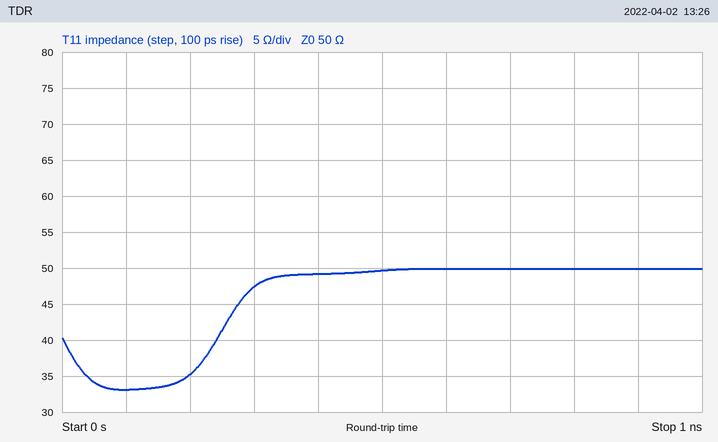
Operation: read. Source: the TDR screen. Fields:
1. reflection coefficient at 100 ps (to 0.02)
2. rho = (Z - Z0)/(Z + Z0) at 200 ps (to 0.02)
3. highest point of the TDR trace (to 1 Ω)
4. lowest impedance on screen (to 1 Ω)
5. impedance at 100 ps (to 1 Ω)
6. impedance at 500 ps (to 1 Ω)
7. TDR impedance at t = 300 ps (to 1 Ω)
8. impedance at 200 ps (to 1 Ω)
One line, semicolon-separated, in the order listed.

-0.20; -0.18; 50 Ω; 33 Ω; 33 Ω; 50 Ω; 47 Ω; 35 Ω
